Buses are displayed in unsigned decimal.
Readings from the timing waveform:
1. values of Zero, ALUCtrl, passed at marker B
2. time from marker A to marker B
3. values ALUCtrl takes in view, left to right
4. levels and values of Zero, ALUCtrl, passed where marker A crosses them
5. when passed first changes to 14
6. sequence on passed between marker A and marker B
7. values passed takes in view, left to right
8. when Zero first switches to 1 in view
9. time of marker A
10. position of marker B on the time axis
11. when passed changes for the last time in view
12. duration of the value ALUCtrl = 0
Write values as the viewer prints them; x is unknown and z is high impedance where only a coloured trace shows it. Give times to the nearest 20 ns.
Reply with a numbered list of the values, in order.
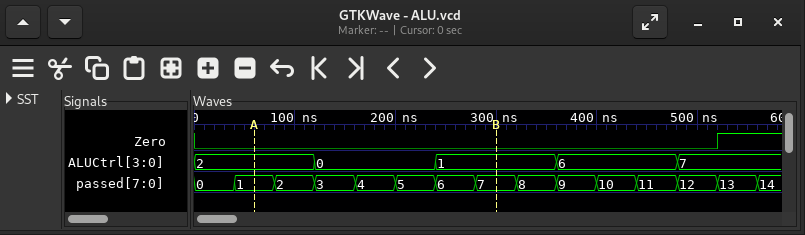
1. Zero=0, ALUCtrl=1, passed=7
2. 240 ns
3. 2, 0, 1, 6, 7
4. Zero=0, ALUCtrl=2, passed=1
5. 560 ns
6. 1, 2, 3, 4, 5, 6, 7
7. 0, 1, 2, 3, 4, 5, 6, 7, 8, 9, 10, 11, 12, 13, 14
8. 520 ns
9. 60 ns
10. 300 ns
11. 560 ns
12. 120 ns
